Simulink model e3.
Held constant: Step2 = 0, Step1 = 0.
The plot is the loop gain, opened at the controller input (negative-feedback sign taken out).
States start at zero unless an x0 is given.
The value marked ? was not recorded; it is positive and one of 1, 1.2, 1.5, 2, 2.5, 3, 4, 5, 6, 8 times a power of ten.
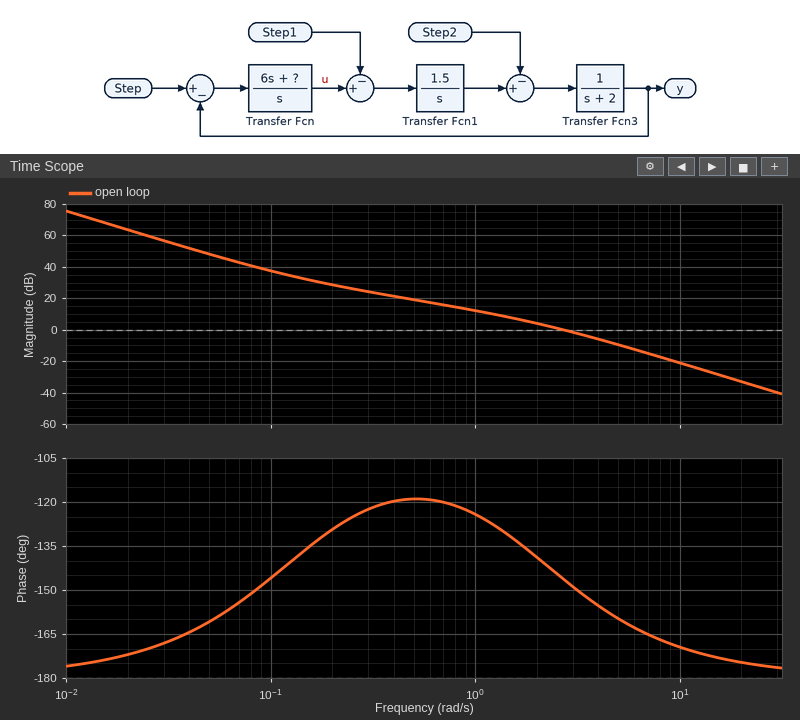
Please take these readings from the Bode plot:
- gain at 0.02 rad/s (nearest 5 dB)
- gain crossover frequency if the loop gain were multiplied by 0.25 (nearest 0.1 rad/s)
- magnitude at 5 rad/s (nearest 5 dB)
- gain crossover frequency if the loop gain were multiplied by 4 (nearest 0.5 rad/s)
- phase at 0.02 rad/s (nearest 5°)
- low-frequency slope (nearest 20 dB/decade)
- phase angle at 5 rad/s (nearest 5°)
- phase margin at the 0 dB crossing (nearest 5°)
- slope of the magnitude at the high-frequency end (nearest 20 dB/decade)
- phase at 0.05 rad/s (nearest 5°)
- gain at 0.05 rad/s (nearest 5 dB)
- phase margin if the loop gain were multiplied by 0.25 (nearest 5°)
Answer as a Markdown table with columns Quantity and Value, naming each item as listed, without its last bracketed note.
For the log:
| Quantity | Value |
|---|---|
| gain at 0.02 rad/s | 65 dB |
| gain crossover frequency if the loop gain were multiplied by 0.25 | 1.0 rad/s |
| magnitude at 5 rad/s | -10 dB |
| gain crossover frequency if the loop gain were multiplied by 4 | 6.0 rad/s |
| phase at 0.02 rad/s | -170° |
| low-frequency slope | -40 dB/decade |
| phase angle at 5 rad/s | -160° |
| phase margin at the 0 dB crossing | 35° |
| slope of the magnitude at the high-frequency end | -40 dB/decade |
| phase at 0.05 rad/s | -160° |
| gain at 0.05 rad/s | 50 dB |
| phase margin if the loop gain were multiplied by 0.25 | 55° |
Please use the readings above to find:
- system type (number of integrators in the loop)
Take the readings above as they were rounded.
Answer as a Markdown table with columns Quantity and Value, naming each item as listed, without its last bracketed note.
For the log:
| Quantity | Value |
|---|---|
| system type | 2 |
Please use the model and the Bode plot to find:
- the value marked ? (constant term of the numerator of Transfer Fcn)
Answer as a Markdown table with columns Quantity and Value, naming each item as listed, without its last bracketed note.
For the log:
| Quantity | Value |
|---|---|
| the value marked ? | 0.8 |
